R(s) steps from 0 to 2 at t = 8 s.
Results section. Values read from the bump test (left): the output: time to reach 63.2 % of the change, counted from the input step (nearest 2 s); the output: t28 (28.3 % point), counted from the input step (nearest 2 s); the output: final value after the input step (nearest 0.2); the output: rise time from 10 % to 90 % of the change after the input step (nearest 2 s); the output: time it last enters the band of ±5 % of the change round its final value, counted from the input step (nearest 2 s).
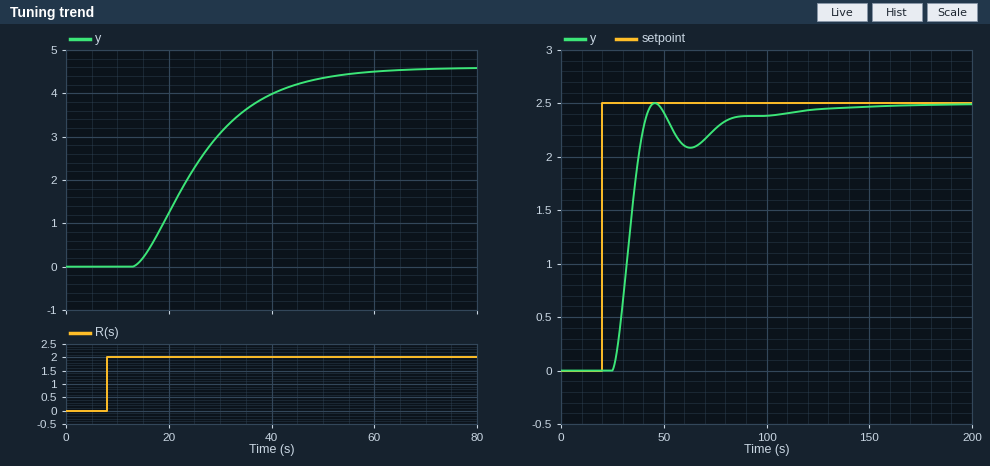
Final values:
20 s
12 s
4.6
26 s
42 s
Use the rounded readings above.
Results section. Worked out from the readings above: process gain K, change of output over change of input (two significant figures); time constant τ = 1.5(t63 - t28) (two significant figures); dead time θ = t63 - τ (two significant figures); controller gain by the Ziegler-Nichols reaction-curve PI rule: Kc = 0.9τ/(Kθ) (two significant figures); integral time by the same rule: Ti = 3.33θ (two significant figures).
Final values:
2.3
12 s
8.0 s
0.59
27 s
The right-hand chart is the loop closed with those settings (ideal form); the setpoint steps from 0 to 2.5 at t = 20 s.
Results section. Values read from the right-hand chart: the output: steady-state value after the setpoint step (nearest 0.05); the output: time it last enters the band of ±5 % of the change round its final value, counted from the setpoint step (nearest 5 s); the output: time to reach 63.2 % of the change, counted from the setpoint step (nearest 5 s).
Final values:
2.50
65 s
15 s
